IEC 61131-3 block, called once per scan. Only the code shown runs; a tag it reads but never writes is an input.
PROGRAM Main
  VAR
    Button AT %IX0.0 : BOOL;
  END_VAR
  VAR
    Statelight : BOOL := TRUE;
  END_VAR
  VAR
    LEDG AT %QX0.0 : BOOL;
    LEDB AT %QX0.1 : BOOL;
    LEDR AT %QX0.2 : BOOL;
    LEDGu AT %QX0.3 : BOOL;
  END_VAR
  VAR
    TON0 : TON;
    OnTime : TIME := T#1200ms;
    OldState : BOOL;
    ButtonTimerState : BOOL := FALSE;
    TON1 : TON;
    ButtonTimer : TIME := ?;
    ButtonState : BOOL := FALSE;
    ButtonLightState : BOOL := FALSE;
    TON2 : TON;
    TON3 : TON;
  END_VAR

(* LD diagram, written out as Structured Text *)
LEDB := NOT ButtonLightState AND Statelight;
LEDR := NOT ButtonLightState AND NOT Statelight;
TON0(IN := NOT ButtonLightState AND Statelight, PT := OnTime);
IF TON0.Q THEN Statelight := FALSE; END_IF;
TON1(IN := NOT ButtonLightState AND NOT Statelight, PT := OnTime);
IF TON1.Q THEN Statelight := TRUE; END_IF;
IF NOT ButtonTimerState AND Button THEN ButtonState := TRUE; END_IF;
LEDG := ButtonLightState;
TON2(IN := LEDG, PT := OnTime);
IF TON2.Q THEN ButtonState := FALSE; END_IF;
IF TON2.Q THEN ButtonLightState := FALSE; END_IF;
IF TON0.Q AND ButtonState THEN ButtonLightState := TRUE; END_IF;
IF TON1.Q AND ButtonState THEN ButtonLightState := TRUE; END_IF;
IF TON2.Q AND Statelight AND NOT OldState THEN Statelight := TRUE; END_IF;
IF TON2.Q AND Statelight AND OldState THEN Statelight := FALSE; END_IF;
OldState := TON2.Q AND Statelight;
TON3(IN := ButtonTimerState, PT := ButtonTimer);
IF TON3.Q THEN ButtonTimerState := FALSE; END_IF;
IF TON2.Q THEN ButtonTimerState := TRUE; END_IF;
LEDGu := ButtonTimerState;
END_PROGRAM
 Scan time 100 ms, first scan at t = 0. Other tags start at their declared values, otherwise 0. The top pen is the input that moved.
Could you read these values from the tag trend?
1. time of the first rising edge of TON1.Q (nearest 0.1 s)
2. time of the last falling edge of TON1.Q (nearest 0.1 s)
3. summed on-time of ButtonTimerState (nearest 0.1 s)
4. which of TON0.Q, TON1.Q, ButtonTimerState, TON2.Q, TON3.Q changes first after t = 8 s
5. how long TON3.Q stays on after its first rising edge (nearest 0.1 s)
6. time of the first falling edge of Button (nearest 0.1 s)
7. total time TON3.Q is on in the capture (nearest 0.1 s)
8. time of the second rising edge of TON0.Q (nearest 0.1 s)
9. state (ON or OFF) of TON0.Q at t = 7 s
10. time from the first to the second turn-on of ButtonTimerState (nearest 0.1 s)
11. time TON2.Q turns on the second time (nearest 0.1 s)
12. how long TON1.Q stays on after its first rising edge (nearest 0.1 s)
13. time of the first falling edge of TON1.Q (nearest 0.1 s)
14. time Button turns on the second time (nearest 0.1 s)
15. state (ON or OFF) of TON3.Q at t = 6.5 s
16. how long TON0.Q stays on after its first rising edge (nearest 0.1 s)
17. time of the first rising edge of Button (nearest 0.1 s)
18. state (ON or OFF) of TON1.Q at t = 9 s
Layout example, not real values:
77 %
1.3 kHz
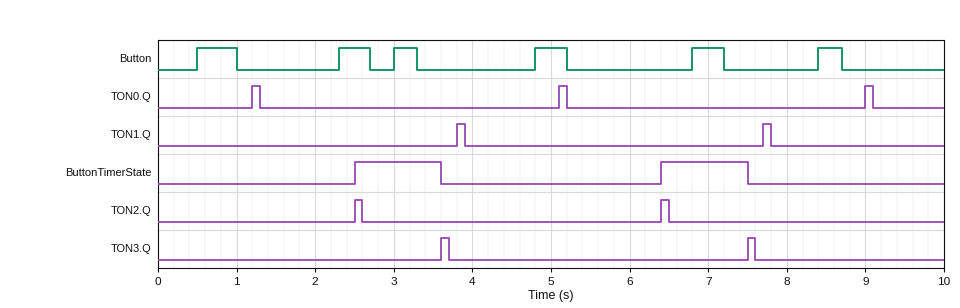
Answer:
3.8 s
7.8 s
2.2 s
TON0.Q
0.1 s
1.0 s
0.2 s
5.1 s
OFF
3.9 s
6.4 s
0.1 s
3.9 s
2.3 s
OFF
0.1 s
0.5 s
OFF
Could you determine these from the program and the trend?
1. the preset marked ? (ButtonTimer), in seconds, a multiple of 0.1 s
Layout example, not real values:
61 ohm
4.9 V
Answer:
1.0 s
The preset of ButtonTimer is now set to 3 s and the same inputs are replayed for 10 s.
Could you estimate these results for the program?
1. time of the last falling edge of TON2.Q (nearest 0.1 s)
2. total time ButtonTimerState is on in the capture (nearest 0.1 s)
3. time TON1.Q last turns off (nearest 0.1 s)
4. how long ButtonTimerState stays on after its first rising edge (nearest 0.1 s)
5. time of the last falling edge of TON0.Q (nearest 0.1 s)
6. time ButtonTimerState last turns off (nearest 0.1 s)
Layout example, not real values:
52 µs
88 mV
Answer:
9.0 s
4.2 s
6.4 s
3.1 s
7.7 s
5.6 s
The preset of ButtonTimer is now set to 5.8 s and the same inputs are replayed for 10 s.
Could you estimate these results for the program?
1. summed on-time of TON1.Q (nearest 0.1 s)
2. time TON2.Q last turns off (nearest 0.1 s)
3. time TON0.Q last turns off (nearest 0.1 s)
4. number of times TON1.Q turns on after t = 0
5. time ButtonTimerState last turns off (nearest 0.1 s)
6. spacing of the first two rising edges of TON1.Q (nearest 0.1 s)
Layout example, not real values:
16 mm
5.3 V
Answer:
0.3 s
2.6 s
7.7 s
3
8.4 s
2.5 s
